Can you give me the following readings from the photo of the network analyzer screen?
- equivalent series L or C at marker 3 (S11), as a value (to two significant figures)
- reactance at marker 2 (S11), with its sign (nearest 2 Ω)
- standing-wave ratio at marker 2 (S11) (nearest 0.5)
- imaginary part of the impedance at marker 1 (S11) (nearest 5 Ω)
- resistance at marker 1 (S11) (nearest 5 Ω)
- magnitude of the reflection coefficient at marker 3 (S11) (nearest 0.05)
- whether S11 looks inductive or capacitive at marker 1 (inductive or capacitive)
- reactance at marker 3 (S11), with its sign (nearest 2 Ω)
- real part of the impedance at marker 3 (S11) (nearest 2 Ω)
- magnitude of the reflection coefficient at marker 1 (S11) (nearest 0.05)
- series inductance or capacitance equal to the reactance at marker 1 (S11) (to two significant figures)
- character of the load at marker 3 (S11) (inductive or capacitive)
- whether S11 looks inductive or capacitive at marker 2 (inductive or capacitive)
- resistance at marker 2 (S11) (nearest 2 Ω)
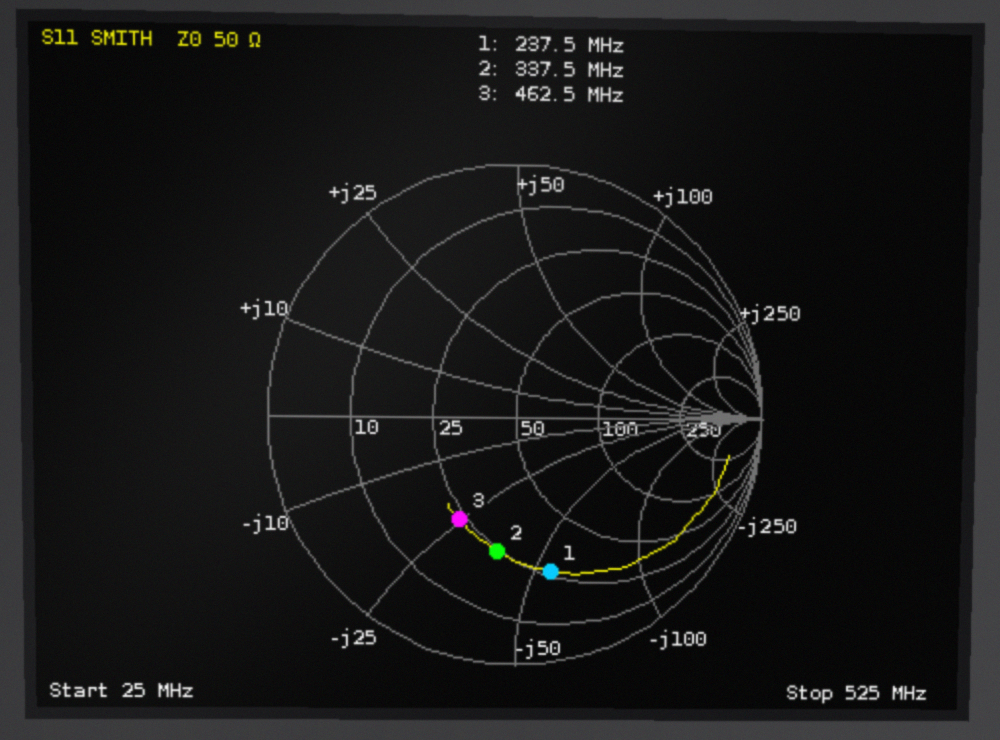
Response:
14 pF
-38 Ω
3.5
-55 Ω
25 Ω
0.45
capacitive
-24 Ω
24 Ω
0.65
12 pF
capacitive
capacitive
24 Ω
